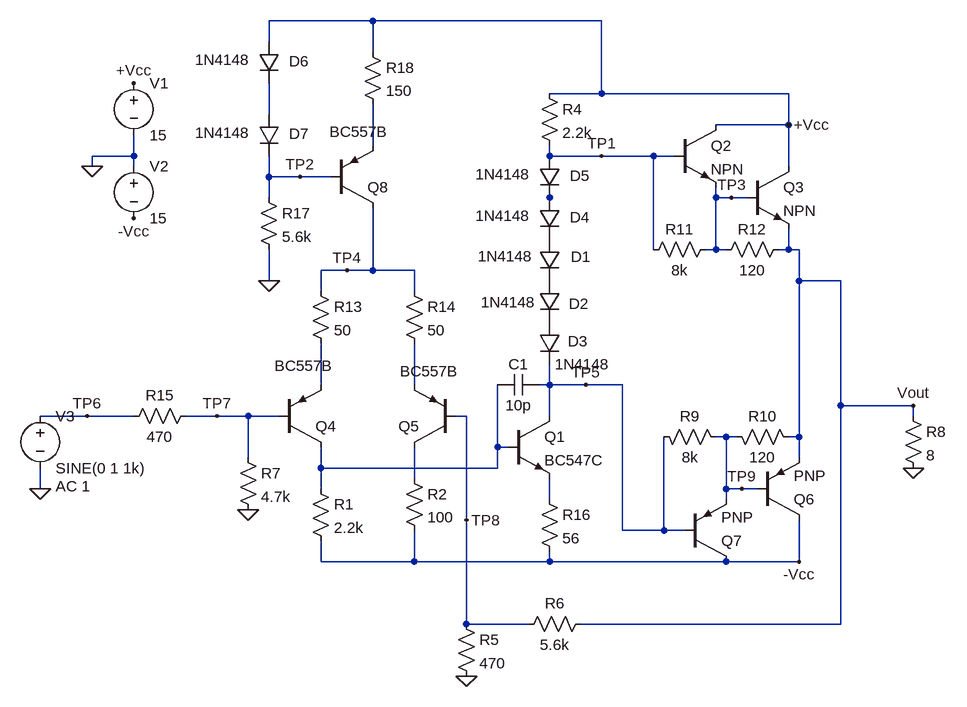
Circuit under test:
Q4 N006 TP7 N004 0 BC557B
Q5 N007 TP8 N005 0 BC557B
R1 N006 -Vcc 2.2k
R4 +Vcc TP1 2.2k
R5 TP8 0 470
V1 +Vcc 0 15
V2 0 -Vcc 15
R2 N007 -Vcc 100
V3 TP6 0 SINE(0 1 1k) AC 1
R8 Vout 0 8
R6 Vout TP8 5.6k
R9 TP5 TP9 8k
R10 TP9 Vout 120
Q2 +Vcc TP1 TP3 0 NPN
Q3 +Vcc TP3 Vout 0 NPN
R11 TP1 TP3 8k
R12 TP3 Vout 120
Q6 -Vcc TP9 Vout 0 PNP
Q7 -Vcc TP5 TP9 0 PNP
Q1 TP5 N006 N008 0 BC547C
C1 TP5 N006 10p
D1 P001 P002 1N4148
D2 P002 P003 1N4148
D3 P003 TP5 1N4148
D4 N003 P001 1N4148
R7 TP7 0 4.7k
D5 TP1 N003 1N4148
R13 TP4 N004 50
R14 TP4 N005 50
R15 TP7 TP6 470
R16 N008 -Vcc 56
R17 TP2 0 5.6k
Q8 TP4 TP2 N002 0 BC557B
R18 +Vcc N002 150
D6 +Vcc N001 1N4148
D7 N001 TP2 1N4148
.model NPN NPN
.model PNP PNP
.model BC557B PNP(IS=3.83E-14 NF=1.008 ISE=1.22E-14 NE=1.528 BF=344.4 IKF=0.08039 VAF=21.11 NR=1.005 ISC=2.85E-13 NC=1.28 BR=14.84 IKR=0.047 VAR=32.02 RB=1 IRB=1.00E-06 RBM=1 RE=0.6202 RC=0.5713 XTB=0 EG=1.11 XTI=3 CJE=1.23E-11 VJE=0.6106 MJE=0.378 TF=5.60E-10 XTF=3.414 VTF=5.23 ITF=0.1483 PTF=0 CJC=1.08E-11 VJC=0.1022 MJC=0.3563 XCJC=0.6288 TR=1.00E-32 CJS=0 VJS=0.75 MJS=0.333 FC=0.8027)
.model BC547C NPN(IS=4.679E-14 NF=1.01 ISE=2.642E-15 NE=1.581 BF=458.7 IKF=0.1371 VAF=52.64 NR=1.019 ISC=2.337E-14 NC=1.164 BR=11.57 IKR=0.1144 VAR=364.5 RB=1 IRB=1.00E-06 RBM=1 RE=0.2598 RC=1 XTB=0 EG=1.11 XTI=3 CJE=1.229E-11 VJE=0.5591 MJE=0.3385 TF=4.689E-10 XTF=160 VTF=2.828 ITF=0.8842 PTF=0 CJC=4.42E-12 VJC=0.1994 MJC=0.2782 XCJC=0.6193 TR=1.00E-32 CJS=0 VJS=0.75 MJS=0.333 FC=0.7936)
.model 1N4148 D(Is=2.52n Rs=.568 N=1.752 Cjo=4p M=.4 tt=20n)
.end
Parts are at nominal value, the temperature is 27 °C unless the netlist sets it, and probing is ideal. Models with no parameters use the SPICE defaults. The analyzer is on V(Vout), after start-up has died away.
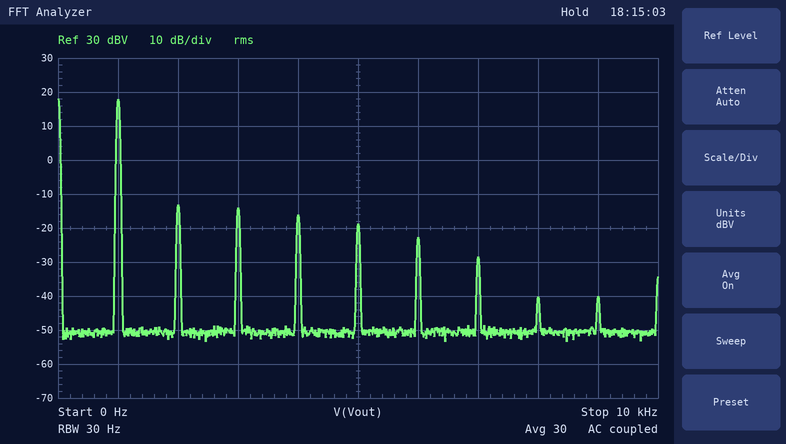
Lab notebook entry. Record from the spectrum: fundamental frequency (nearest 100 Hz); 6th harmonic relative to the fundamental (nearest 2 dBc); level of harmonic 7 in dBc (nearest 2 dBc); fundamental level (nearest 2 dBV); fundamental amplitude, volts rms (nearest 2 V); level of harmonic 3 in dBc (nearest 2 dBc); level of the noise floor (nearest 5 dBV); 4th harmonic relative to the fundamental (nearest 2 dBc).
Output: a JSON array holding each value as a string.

["1.0 kHz", "-40 dBc", "-46 dBc", "18 dBV", "8 V", "-32 dBc", "-50 dBV", "-34 dBc"]
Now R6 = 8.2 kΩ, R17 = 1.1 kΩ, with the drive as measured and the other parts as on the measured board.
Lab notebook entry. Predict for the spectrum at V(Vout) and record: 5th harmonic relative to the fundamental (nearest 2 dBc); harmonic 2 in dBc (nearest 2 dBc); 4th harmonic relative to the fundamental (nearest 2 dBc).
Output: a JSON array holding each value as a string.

["-34 dBc", "-14 dBc", "-38 dBc"]
